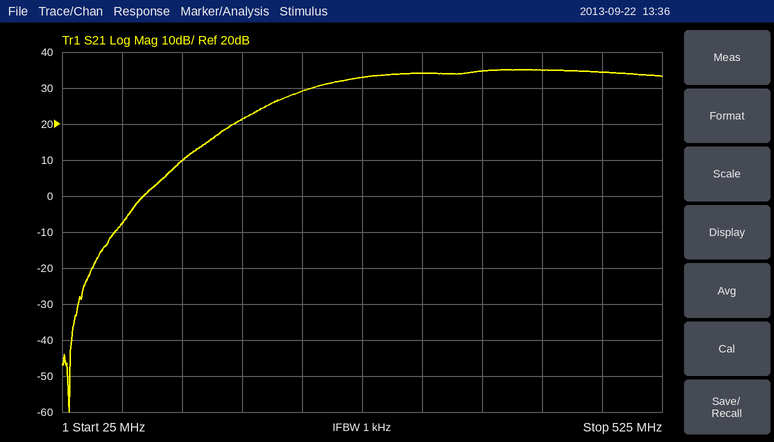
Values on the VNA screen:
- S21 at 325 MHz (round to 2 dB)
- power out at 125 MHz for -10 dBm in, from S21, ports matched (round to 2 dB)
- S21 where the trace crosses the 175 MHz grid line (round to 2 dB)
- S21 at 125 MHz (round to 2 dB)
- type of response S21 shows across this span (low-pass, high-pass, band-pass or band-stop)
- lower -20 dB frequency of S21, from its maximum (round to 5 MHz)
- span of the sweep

34 dB
0 dBm
22 dB
10 dB
high-pass
145 MHz
500 MHz
